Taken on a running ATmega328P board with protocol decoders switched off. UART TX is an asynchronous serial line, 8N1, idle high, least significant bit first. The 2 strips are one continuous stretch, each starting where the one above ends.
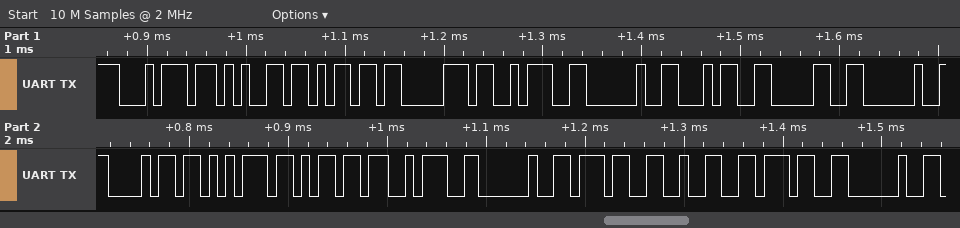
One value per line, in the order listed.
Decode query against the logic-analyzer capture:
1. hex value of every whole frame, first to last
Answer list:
0x74 0x65 0x6D 0x70 0x3A 0x20 0x34 0x30 0x20 0x68 0x75 0x6D 0x3A 0x20 0x37 0x32 0x37 0x20
